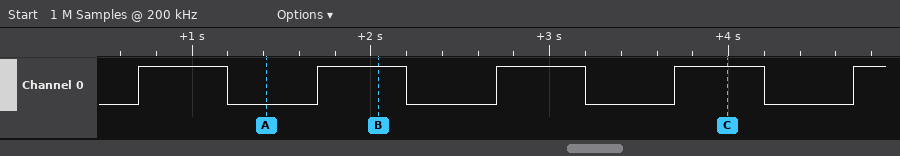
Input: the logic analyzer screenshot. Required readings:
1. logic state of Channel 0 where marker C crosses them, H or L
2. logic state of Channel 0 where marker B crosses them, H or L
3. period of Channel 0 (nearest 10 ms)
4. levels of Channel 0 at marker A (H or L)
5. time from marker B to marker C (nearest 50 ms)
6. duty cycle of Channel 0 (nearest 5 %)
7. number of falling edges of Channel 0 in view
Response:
Channel 0=H
Channel 0=H
1000 ms
Channel 0=L
1950 ms
50 %
4
